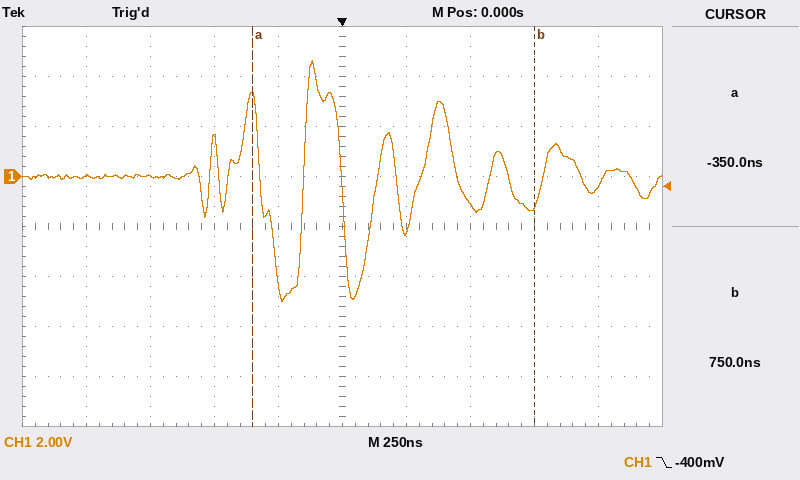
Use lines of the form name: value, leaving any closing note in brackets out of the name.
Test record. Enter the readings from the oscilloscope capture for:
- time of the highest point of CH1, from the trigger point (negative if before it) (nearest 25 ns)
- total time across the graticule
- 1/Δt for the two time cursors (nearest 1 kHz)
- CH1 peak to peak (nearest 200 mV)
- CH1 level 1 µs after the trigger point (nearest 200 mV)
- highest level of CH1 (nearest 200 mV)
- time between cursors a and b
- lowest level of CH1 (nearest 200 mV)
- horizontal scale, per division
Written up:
time of the highest point of CH1, from the trigger point (negative if before it): -125 ns
total time across the graticule: 2.5 µs
1/Δt for the two time cursors: 909 kHz
CH1 peak to peak: 9.6 V
CH1 level 1 µs after the trigger point: -400 mV
highest level of CH1: 4.6 V
time between cursors a and b: 1.100 µs
lowest level of CH1: -5.0 V
horizontal scale, per division: 250 ns
